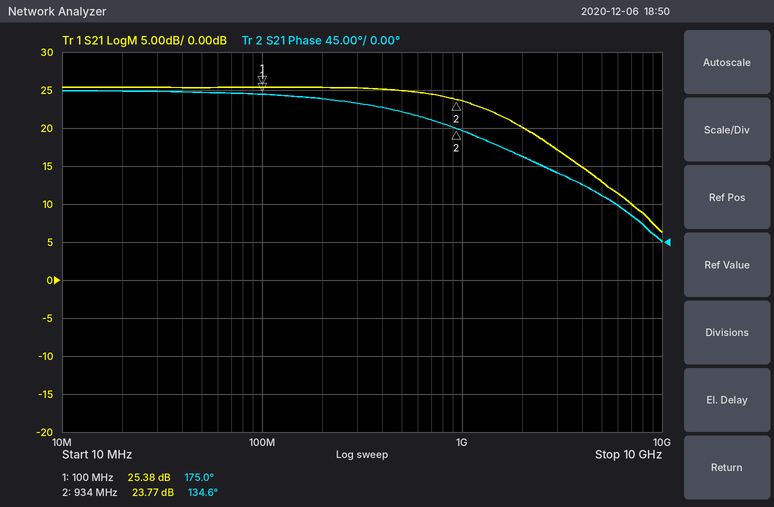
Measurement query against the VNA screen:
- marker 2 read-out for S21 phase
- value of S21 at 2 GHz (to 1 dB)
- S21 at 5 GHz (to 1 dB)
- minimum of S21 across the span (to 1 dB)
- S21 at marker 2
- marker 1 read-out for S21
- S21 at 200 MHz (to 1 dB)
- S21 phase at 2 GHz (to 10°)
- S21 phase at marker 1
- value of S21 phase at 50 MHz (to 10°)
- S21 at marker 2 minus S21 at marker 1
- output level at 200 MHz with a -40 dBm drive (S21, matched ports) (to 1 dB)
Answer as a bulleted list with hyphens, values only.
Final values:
- 134.6°
- 20 dB
- 13 dB
- 6 dB
- 23.77 dB
- 25.38 dB
- 25 dB
- 100°
- 175.0°
- 180°
- -1.61 dB
- -15 dBm
